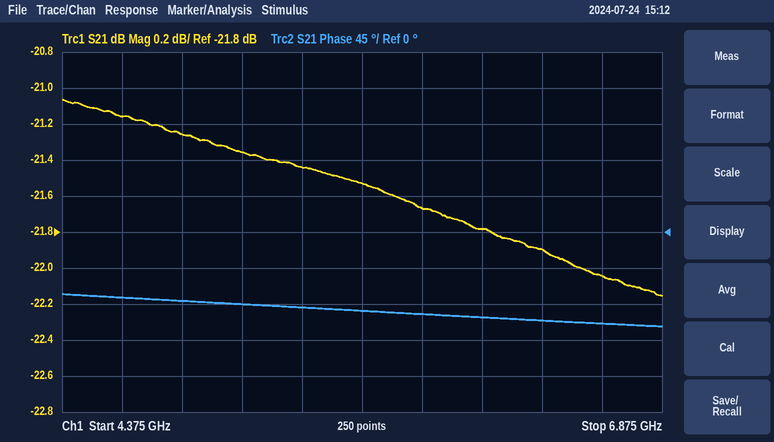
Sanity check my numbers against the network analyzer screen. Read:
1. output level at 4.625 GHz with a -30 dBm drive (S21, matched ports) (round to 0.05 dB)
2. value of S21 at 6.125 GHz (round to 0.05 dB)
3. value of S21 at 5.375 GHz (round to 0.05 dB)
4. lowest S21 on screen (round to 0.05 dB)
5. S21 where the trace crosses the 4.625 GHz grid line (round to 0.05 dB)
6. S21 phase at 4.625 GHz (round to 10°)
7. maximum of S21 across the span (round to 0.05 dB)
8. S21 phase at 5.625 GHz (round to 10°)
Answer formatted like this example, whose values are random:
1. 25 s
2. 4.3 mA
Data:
1. -51.15 dBm
2. -21.80 dB
3. -21.45 dB
4. -22.15 dB
5. -21.15 dB
6. -80°
7. -21.05 dB
8. -100°
